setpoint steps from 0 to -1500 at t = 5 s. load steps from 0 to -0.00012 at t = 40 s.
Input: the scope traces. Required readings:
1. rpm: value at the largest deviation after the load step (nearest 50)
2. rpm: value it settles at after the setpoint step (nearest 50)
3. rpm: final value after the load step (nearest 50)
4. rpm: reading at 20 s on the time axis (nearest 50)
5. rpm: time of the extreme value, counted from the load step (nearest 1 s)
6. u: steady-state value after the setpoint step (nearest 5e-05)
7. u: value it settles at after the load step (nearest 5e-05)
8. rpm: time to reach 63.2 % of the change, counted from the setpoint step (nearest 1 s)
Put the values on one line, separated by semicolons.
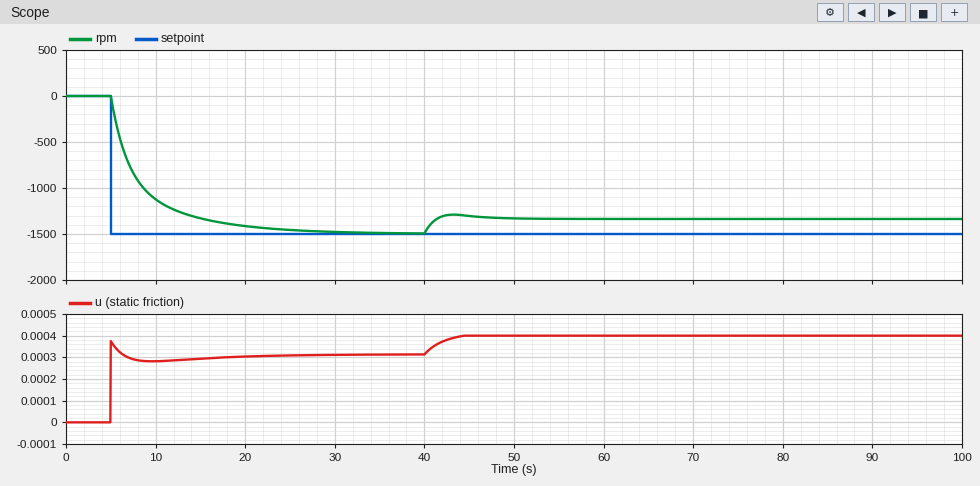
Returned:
-1300; -1500; -1350; -1400; 3 s; 0.00030; 0.00040; 3 s
